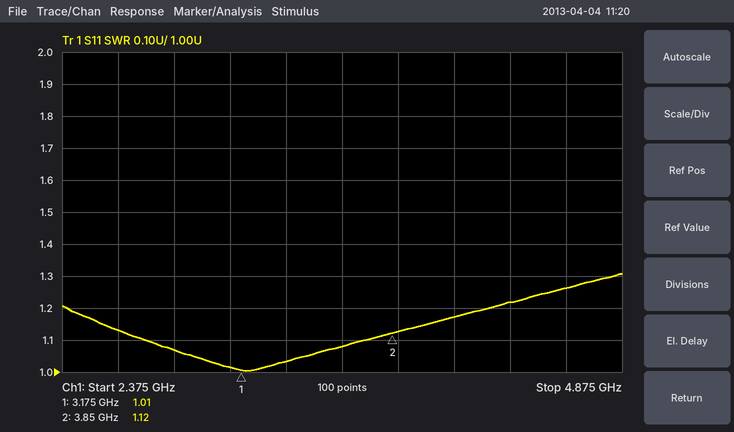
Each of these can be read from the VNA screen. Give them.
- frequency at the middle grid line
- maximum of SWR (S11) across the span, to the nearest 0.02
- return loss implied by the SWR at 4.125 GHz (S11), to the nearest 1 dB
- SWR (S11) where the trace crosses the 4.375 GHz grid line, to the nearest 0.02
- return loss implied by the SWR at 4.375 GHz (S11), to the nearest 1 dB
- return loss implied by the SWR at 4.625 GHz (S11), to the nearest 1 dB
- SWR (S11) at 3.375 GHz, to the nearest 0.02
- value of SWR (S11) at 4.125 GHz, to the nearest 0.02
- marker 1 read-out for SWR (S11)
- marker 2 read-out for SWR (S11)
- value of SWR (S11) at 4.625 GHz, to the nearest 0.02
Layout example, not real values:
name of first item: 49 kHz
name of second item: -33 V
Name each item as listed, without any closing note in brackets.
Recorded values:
frequency at the middle grid line: 3.625 GHz
maximum of SWR (S11) across the span, to the nearest 0.02: 1.30
return loss implied by the SWR at 4.125 GHz (S11), to the nearest 1 dB: 22 dB
SWR (S11) where the trace crosses the 4.375 GHz grid line, to the nearest 0.02: 1.22
return loss implied by the SWR at 4.375 GHz (S11), to the nearest 1 dB: 20 dB
return loss implied by the SWR at 4.625 GHz (S11), to the nearest 1 dB: 19 dB
SWR (S11) at 3.375 GHz, to the nearest 0.02: 1.04
value of SWR (S11) at 4.125 GHz, to the nearest 0.02: 1.18
marker 1 read-out for SWR: 1.01
marker 2 read-out for SWR: 1.12
value of SWR (S11) at 4.625 GHz, to the nearest 0.02: 1.26
